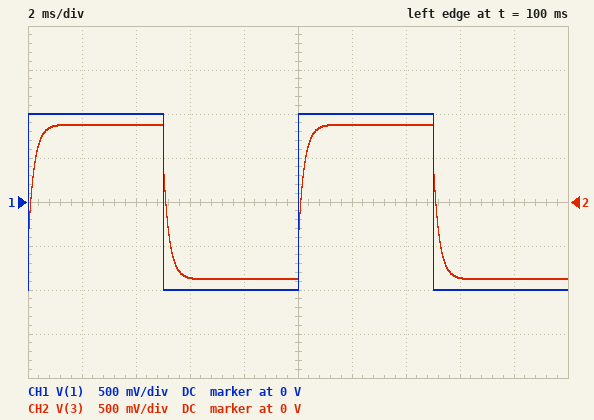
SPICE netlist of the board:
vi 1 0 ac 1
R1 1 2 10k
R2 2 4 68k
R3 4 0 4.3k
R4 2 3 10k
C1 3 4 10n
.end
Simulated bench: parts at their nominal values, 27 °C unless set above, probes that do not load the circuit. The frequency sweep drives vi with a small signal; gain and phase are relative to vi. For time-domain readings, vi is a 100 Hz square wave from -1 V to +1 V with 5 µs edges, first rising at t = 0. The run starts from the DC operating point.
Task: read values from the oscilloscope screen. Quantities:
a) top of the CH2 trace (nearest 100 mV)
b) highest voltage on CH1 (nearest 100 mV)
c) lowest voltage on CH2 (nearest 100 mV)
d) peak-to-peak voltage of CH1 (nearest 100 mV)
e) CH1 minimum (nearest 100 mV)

900 mV
1.0 V
-900 mV
2.0 V
-1.0 V
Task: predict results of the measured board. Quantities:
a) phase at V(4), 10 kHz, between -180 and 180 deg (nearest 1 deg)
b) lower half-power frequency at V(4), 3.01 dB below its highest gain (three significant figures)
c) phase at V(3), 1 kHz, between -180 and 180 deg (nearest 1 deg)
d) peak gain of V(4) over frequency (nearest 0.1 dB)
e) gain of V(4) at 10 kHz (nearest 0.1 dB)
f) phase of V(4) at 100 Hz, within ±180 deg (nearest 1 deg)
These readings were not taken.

3 deg
670 Hz
-38 deg
-14.6 dB
-14.6 dB
18 deg
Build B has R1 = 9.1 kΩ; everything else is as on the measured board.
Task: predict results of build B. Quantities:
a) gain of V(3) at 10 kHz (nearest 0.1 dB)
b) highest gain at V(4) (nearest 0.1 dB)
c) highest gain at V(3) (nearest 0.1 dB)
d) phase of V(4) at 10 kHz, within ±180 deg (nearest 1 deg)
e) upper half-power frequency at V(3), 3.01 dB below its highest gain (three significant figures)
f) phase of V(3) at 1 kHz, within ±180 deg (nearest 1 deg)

-13.8 dB
-14.2 dB
-1.0 dB
3 deg
790 Hz
-37 deg
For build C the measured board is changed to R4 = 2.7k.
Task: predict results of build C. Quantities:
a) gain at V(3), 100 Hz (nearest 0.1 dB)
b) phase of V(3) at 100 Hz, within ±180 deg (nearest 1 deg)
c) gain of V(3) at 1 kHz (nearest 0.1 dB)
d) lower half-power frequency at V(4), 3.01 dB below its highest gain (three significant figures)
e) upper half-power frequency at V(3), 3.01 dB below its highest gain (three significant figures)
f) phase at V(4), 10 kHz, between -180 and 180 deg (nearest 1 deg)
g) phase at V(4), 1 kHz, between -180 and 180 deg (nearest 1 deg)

-1.2 dB
-4 deg
-3.5 dB
1.05 kHz
1.20 kHz
5 deg
35 deg
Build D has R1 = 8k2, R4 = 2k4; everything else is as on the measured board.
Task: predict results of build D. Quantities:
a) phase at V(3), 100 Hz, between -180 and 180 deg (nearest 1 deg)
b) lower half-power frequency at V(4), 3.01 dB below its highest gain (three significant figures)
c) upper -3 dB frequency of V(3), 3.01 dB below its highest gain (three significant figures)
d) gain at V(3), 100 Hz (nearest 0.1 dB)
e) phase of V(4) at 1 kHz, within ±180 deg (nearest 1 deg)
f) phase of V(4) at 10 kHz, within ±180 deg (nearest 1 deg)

-3 deg
1.19 kHz
1.38 kHz
-1.0 dB
38 deg
6 deg
